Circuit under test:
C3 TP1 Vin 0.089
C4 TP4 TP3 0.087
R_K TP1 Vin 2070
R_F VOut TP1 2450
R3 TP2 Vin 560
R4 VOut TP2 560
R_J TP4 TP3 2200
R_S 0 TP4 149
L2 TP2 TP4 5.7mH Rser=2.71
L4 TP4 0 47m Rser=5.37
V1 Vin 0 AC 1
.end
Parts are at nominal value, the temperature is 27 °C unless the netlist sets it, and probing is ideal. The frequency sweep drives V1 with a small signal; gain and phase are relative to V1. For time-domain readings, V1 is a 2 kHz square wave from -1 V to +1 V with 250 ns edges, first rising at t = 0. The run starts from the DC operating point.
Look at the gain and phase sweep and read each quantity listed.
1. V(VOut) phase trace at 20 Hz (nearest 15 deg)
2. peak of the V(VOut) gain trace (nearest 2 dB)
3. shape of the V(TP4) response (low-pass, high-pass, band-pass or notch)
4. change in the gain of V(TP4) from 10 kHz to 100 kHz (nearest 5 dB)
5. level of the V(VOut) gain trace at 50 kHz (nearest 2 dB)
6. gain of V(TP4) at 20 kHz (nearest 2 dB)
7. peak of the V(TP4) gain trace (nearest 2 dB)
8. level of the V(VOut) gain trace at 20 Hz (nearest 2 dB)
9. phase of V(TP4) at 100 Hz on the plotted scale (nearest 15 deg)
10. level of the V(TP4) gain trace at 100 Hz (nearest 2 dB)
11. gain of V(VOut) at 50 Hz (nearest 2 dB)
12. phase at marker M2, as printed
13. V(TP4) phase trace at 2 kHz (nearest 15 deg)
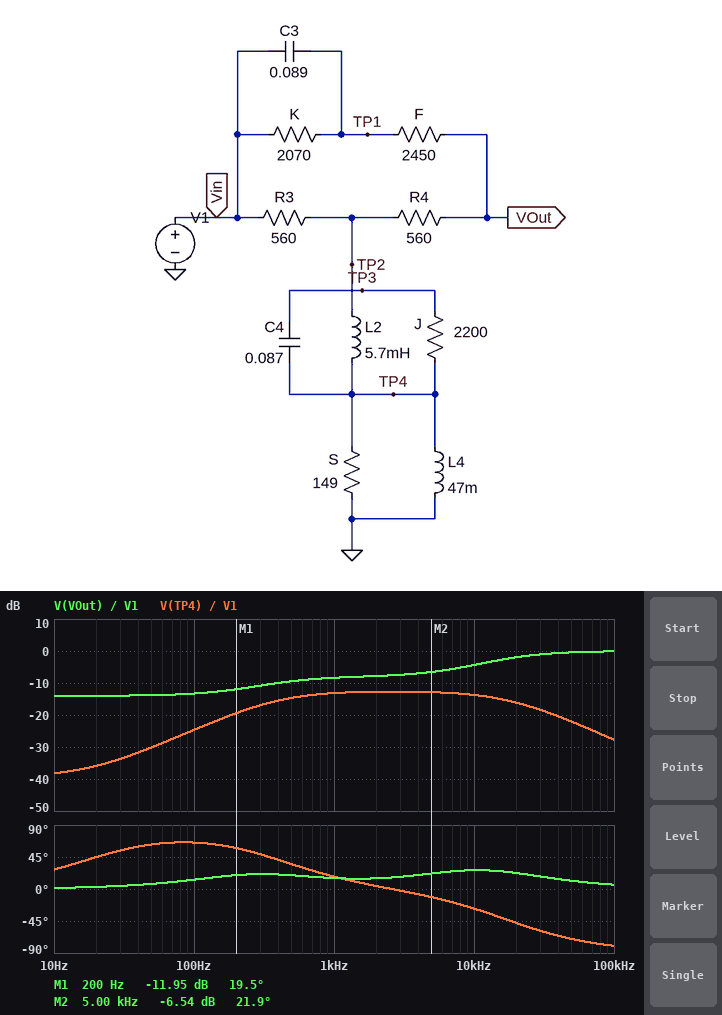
0 deg
0 dB
band-pass
-15 dB
0 dB
-16 dB
-12 dB
-14 dB
60 deg
-24 dB
-14 dB
21.9 deg
0 deg
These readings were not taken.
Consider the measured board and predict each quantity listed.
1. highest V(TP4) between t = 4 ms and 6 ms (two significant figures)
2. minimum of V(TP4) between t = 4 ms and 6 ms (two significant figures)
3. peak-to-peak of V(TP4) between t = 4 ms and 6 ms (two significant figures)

280 mV
-280 mV
560 mV
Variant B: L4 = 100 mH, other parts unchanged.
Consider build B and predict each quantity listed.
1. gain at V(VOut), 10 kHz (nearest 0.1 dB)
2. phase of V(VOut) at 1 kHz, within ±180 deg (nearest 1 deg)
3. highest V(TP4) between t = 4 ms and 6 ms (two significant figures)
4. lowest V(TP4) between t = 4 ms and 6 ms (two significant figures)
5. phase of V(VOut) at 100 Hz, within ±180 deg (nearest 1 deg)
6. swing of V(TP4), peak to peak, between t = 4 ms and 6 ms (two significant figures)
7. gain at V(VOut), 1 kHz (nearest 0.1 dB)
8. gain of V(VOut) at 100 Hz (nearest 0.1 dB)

-4.4 dB
10 deg
260 mV
-260 mV
19 deg
520 mV
-8.2 dB
-11.9 dB
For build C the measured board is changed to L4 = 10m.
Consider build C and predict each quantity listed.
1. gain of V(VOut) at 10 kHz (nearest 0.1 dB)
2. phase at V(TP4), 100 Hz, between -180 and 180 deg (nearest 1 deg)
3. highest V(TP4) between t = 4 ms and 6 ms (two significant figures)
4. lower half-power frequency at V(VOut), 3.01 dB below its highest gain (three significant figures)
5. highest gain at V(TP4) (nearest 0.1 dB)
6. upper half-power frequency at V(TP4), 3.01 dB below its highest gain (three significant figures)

-4.1 dB
46 deg
330 mV
13.9 kHz
-13.6 dB
21.4 kHz
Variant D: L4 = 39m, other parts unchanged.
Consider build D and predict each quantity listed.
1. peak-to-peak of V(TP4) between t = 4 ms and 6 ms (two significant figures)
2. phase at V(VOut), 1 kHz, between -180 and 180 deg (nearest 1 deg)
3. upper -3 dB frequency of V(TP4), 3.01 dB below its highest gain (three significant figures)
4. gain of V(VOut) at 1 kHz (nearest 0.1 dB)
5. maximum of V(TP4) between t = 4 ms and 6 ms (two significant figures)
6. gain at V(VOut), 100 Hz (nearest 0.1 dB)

570 mV
17 deg
18.5 kHz
-8.5 dB
290 mV
-13.5 dB
